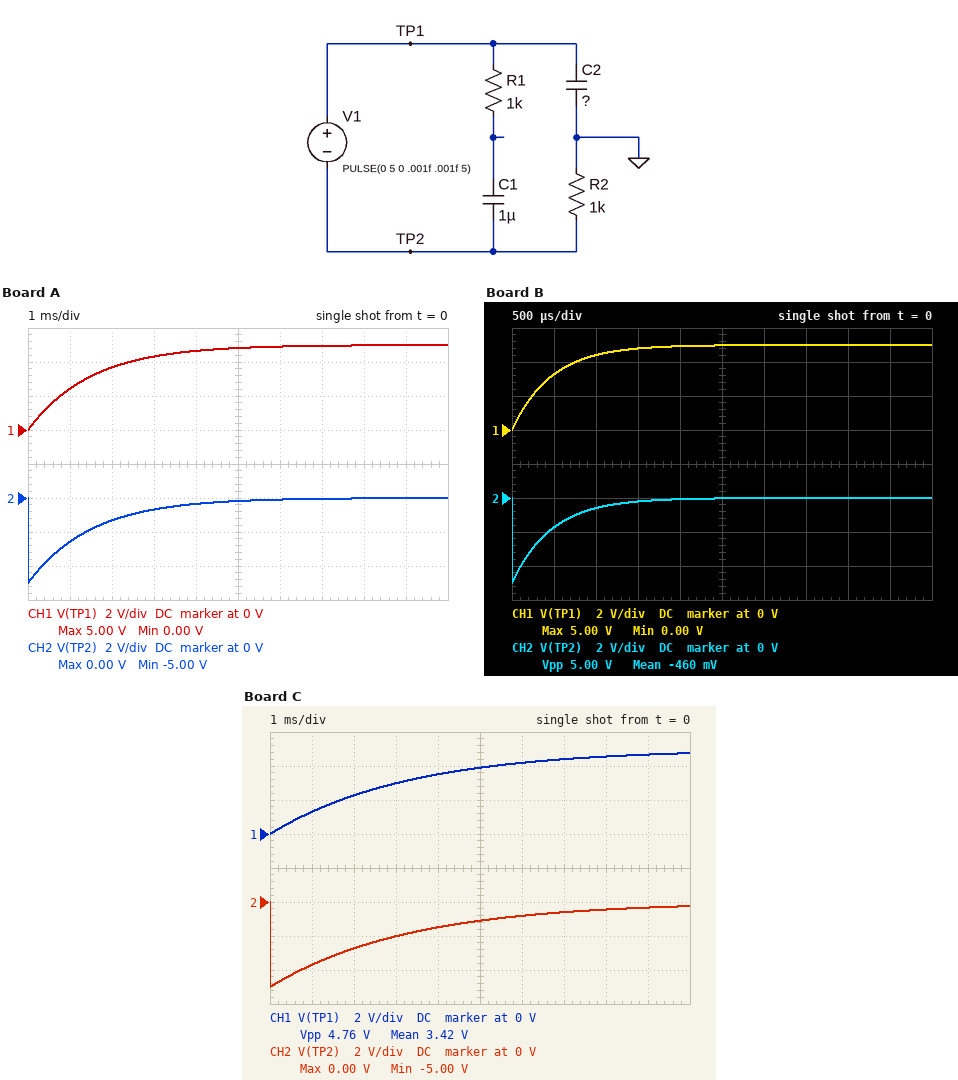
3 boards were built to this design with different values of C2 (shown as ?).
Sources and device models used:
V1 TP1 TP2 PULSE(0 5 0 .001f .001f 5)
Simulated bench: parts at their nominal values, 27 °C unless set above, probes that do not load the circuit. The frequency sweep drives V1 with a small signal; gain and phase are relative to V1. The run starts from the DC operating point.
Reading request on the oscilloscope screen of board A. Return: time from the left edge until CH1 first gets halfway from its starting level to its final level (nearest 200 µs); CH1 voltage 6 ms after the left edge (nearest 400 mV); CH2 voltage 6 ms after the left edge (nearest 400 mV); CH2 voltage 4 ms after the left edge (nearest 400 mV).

1.0 ms
4.8 V
0 V
-400 mV
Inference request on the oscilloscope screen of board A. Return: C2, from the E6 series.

1.5 µF
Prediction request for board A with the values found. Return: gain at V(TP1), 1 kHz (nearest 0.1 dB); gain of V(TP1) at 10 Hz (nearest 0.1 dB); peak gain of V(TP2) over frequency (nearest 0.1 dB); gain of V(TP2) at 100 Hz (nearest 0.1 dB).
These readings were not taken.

-19.5 dB
0 dB
0 dB
-3.3 dB
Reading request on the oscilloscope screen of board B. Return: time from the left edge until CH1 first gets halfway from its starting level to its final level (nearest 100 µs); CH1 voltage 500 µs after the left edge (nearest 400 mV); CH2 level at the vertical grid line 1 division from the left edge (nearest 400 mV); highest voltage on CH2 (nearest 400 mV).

300 µs
3.2 V
-1.6 V
0 V
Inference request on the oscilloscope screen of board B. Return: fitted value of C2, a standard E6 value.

470 nF
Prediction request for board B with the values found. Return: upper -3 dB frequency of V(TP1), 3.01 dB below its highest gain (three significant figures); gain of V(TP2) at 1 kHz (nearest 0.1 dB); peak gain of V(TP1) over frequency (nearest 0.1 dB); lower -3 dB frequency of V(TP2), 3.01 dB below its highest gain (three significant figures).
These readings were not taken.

339 Hz
-0.5 dB
0 dB
339 Hz
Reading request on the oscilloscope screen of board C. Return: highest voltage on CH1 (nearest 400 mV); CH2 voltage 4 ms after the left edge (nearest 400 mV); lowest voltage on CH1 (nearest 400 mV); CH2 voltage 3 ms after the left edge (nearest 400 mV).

4.8 V
-1.6 V
0 V
-2.0 V
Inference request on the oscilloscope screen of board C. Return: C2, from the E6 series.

3.3 µF
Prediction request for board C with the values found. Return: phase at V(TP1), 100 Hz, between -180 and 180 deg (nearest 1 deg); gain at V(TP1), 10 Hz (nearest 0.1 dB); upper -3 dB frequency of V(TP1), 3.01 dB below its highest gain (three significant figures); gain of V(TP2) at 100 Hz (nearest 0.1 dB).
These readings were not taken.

-64 deg
-0.2 dB
48.2 Hz
-0.9 dB
